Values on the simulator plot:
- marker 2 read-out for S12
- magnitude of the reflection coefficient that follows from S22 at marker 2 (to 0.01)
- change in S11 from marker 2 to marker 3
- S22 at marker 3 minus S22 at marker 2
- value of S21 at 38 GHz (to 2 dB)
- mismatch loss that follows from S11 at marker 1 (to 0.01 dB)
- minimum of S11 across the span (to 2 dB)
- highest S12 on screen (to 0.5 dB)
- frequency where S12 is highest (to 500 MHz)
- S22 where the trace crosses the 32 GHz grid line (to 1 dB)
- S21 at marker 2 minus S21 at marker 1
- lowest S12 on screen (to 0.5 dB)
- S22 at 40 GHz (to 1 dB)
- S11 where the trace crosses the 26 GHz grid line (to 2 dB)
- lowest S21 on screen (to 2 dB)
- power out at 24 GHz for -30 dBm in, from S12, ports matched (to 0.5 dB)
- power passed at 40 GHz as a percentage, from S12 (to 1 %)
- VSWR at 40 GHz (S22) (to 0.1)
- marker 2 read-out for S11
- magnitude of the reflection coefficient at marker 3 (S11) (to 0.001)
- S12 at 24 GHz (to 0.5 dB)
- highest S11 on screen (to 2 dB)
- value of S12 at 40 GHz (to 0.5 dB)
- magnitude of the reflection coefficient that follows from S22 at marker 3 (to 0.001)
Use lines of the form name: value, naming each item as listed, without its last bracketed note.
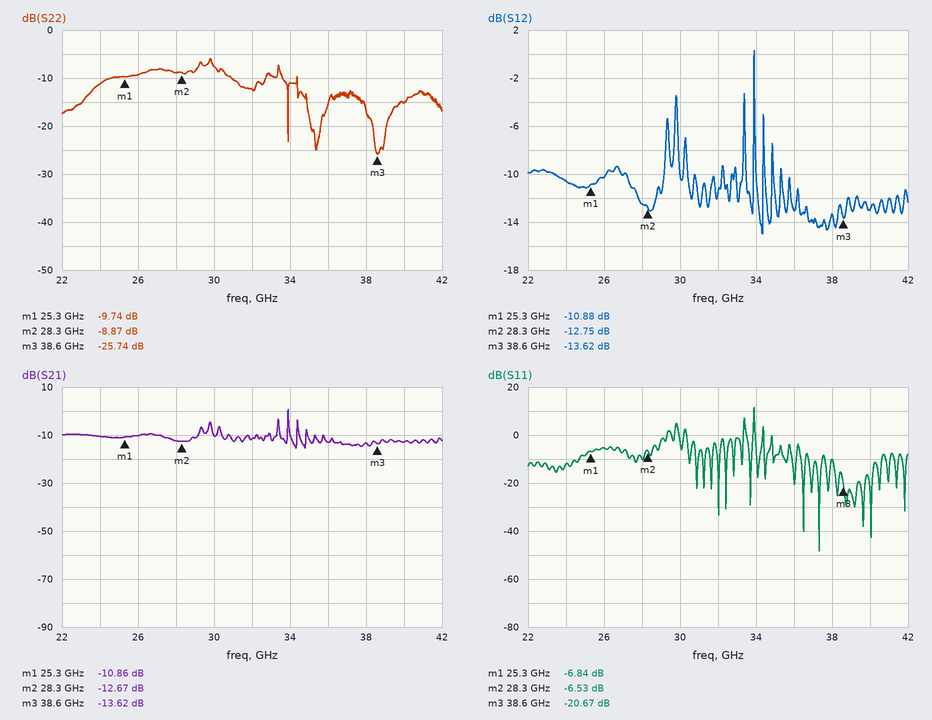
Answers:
marker 2 read-out for S12: -12.75 dB
magnitude of the reflection coefficient that follows from S22 at marker 2: 0.36
change in S11 from marker 2 to marker 3: -14.14 dB
S22 at marker 3 minus S22 at marker 2: -16.87 dB
value of S21 at 38 GHz: -14 dB
mismatch loss that follows from S11 at marker 1: 1.01 dB
minimum of S11 across the span: -48 dB
highest S12 on screen: 0.5 dB
frequency where S12 is highest: 34.0 GHz
S22 where the trace crosses the 32 GHz grid line: -12 dB
S21 at marker 2 minus S21 at marker 1: -1.81 dB
lowest S12 on screen: -15.0 dB
S22 at 40 GHz: -15 dB
S11 where the trace crosses the 26 GHz grid line: -6 dB
lowest S21 on screen: -16 dB
power out at 24 GHz for -30 dBm in, from S12, ports matched: -40.5 dBm
power passed at 40 GHz as a percentage, from S12: 5 %
VSWR at 40 GHz (S22): 1.4
marker 2 read-out for S11: -6.53 dB
magnitude of the reflection coefficient at marker 3 (S11): 0.093
S12 at 24 GHz: -10.5 dB
highest S11 on screen: 12 dB
value of S12 at 40 GHz: -13.0 dB
magnitude of the reflection coefficient that follows from S22 at marker 3: 0.052
